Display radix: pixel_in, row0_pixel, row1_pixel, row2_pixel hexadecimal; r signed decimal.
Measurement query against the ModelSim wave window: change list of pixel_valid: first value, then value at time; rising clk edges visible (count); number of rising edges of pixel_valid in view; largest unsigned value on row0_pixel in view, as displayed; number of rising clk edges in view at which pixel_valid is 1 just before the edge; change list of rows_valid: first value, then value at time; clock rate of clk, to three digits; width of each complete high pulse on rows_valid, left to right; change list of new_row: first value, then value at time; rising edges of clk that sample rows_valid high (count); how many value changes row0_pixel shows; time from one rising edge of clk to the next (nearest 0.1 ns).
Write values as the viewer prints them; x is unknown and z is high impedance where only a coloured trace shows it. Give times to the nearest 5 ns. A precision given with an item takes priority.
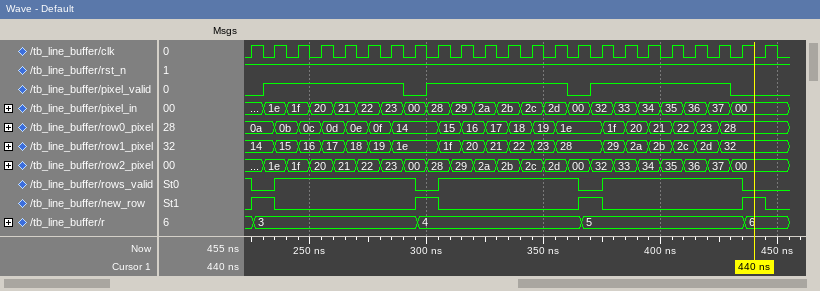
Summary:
0, 1 at 230 ns, 0 at 290 ns, 1 at 300 ns, 0 at 360 ns, 1 at 370 ns, 0 at 430 ns
23
3
28
18
1, 0 at 225 ns, 1 at 235 ns, 0 at 295 ns, 1 at 305 ns, 0 at 365 ns, 1 at 375 ns, 0 at 435 ns
100 MHz
60 ns, 60 ns, 60 ns
0, 1 at 225 ns, 0 at 235 ns, 1 at 295 ns, 0 at 305 ns, 1 at 365 ns, 0 at 375 ns, 1 at 435 ns, 0 at 445 ns
19
18
10 ns
